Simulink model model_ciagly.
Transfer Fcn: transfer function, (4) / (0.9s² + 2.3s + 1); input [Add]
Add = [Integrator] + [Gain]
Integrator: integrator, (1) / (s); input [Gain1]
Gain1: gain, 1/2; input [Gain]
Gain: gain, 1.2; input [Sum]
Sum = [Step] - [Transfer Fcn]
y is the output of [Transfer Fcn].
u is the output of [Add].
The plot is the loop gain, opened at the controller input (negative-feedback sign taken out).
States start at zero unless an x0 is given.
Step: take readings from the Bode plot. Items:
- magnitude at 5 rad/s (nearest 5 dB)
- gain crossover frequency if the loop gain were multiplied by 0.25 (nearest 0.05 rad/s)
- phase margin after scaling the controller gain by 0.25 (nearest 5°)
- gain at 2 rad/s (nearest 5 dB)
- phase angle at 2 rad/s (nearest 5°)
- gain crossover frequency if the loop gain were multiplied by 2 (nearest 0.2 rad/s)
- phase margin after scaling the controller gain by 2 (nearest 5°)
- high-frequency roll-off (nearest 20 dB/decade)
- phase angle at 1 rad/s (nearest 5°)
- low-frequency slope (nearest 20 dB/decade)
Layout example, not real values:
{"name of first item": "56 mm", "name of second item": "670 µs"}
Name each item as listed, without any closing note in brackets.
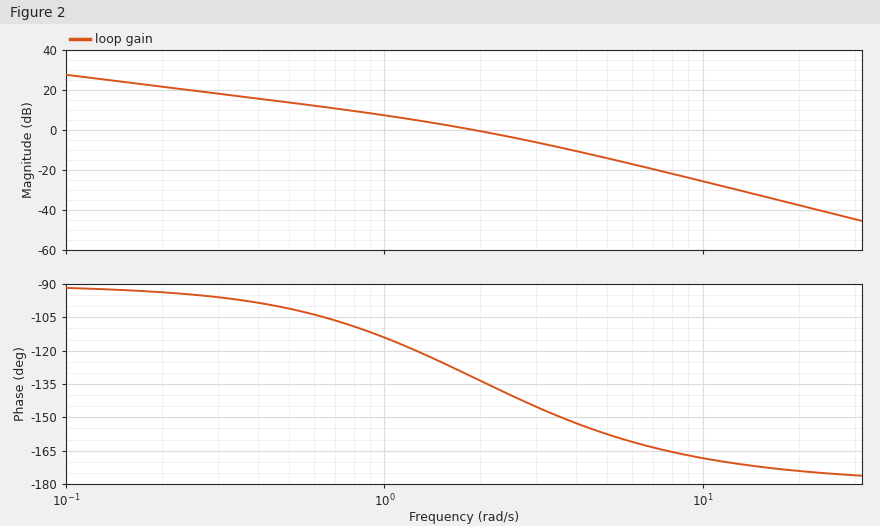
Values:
{"magnitude at 5 rad/s": "-15 dB", "gain crossover frequency if the loop gain were multiplied by 0.25": "0.60 rad/s", "phase margin after scaling the controller gain by 0.25": "75°", "gain at 2 rad/s": "0 dB", "phase angle at 2 rad/s": "-135°", "gain crossover frequency if the loop gain were multiplied by 2": "3.0 rad/s", "phase margin after scaling the controller gain by 2": "35°", "high-frequency roll-off": "-40 dB/decade", "phase angle at 1 rad/s": "-115°", "low-frequency slope": "-20 dB/decade"}
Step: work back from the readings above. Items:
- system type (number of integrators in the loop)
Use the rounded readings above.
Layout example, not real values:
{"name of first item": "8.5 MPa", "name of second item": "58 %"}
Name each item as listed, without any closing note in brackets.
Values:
{"system type": "1"}
